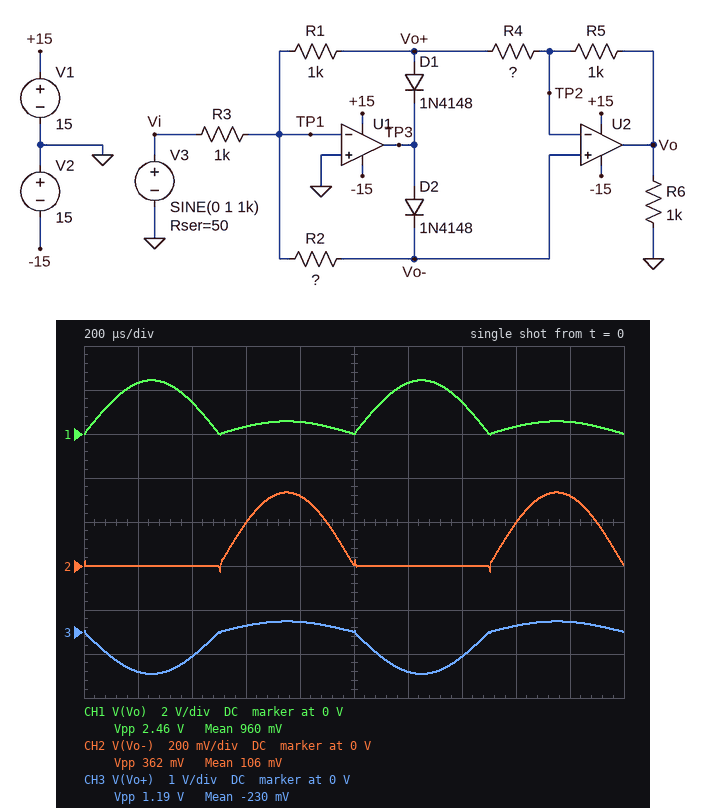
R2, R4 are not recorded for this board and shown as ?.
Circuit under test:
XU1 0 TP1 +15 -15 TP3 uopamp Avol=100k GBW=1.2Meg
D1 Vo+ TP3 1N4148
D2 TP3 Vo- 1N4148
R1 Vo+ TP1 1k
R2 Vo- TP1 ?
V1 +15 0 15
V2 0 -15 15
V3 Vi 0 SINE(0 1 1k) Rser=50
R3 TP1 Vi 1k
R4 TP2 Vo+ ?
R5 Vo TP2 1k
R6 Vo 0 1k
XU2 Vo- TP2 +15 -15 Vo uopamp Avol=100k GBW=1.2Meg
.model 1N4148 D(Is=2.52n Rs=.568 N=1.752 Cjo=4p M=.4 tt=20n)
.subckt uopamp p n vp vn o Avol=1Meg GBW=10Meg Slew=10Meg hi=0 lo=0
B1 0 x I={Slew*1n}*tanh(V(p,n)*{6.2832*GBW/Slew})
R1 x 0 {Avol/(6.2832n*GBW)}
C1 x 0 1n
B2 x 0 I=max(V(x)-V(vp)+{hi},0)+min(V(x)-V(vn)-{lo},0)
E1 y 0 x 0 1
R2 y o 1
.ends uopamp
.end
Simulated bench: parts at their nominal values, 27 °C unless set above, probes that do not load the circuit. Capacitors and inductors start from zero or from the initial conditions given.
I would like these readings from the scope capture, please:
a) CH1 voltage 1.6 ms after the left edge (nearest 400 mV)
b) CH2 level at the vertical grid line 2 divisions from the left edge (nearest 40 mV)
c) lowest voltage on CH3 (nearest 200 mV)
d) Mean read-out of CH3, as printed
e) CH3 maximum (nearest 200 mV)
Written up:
400 mV
0 V
-1.0 V
-230 mV
200 mV
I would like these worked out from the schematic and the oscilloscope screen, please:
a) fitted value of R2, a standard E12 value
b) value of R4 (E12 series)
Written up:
470 Ω
390 Ω
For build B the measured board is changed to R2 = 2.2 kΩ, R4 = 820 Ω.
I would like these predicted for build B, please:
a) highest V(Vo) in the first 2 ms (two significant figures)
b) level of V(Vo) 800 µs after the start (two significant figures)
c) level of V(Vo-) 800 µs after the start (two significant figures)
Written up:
1.5 V
1.4 V
900 mV
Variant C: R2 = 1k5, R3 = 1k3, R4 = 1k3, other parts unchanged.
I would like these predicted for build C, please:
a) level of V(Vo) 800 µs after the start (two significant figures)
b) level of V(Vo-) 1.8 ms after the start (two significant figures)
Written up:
920 mV
640 mV
